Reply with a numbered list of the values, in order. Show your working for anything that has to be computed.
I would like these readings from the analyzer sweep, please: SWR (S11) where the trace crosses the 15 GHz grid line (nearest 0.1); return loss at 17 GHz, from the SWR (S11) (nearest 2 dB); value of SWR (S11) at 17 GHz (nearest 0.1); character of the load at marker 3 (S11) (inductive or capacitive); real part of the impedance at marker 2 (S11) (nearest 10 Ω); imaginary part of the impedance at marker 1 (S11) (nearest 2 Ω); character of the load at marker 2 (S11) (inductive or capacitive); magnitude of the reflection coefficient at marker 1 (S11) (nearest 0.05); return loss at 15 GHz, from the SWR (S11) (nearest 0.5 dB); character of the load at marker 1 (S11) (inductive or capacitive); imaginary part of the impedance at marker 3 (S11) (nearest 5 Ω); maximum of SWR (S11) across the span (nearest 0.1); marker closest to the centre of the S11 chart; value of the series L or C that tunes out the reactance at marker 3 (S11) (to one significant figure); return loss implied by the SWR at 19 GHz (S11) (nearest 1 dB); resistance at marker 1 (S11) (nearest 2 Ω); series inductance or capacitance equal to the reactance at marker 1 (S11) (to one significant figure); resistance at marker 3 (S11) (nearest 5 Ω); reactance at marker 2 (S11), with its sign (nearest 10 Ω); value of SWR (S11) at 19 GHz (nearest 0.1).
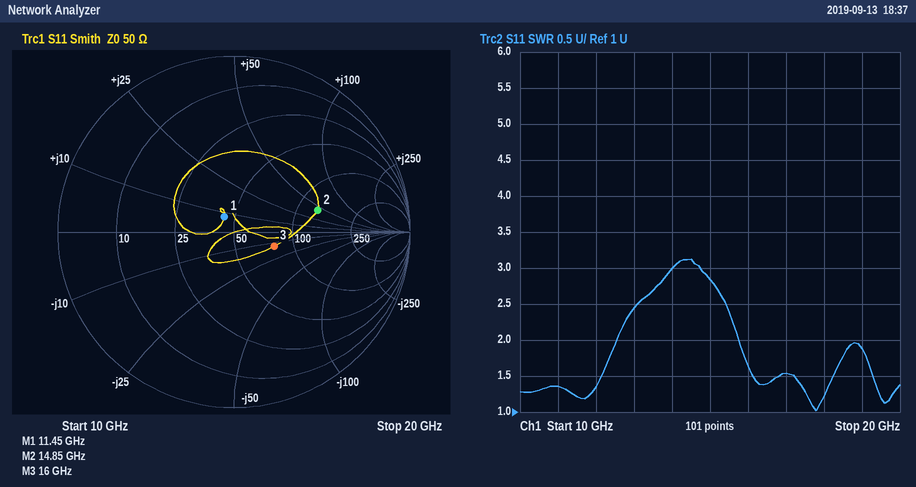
1. 2.8
2. −20 log10((1.5 − 1)/(1.5 + 1)) ≈ 14 dB
3. 1.5
4. capacitive
5. 130 Ω
6. +8 Ω
7. inductive
8. 0.10
9. −20 log10((2.8 − 1)/(2.8 + 1)) ≈ 6.5 dB
10. inductive
11. -15 Ω
12. 3.1
13. marker 1
14. L = 15 Ω/(2π × 16 GHz) ≈ 149 pH, so 100 pH to one significant figure
15. −20 log10((1.9 − 1)/(1.9 + 1)) ≈ 10 dB
16. 44 Ω
17. L = 8 Ω/(2π × 11.45 GHz) ≈ 111 pH, so 100 pH to one significant figure
18. 80 Ω
19. +40 Ω
20. 1.9
